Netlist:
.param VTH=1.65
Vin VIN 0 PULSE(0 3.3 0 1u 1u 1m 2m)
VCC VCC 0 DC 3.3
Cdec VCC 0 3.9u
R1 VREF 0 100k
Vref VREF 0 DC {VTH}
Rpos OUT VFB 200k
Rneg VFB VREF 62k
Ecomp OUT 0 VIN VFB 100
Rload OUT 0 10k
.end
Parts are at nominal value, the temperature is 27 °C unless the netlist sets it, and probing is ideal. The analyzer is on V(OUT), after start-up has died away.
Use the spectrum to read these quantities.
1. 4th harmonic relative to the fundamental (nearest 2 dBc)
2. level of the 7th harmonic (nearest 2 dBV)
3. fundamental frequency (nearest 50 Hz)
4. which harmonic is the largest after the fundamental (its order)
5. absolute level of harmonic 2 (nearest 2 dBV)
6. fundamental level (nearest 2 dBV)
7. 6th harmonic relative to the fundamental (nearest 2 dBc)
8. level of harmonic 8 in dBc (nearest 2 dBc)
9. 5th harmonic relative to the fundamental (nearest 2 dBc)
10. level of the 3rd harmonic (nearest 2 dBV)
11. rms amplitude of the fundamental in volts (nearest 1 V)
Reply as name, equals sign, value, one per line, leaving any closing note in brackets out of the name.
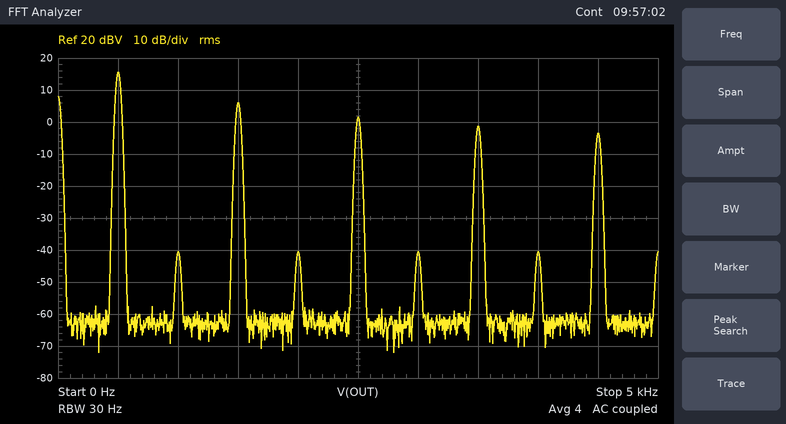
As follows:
4th harmonic relative to the fundamental = -56 dBc
level of the 7th harmonic = -2 dBV
fundamental frequency = 500 Hz
which harmonic is the largest after the fundamental = 3
absolute level of harmonic 2 = -40 dBV
fundamental level = 16 dBV
6th harmonic relative to the fundamental = -56 dBc
level of harmonic 8 in dBc = -56 dBc
5th harmonic relative to the fundamental = -14 dBc
level of the 3rd harmonic = 6 dBV
rms amplitude of the fundamental in volts = 6 V
